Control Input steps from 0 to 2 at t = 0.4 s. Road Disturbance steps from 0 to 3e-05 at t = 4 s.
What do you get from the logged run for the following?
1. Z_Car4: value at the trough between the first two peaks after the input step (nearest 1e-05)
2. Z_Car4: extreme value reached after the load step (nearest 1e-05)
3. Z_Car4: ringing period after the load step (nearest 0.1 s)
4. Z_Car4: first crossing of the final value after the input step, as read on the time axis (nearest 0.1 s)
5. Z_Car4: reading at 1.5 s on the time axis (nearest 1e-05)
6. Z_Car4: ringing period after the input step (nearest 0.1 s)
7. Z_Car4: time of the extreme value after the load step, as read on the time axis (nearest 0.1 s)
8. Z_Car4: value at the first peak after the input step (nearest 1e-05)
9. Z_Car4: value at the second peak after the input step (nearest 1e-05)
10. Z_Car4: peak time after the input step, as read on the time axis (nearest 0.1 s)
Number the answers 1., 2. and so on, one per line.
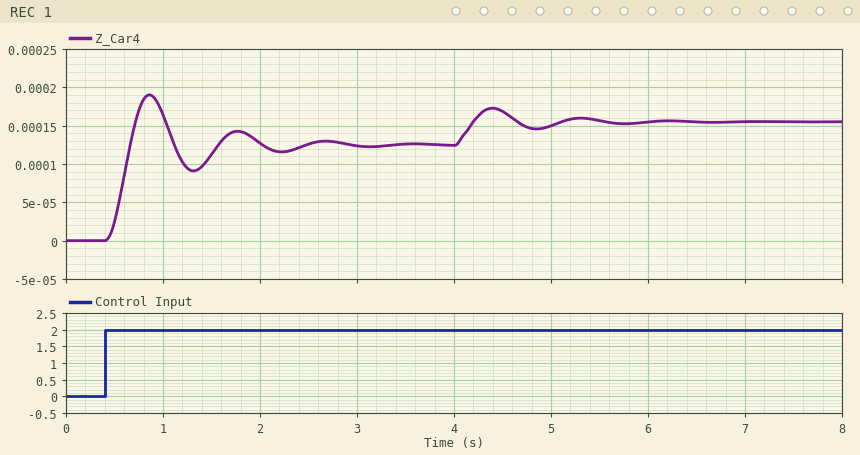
1. 0.00009
2. 0.00017
3. 0.9 s
4. 0.7 s
5. 0.00011
6. 0.9 s
7. 4.4 s
8. 0.00019
9. 0.00014
10. 0.9 s
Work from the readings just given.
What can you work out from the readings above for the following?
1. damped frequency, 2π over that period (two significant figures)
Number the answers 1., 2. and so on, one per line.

1. 7.0 rad/s
